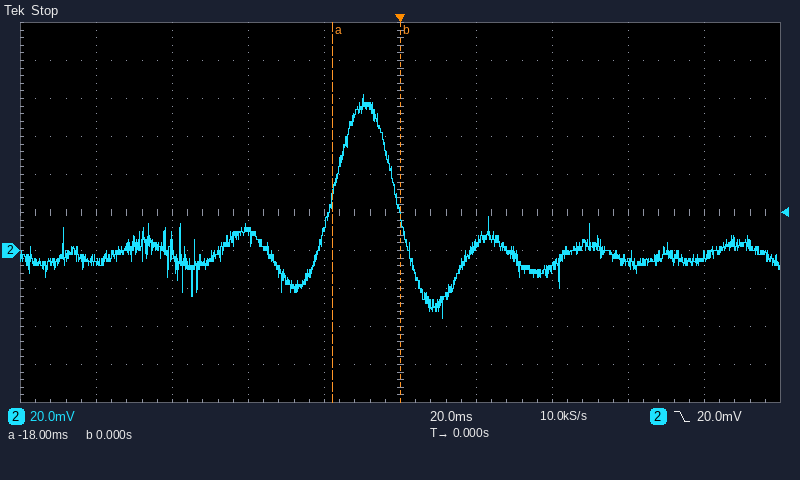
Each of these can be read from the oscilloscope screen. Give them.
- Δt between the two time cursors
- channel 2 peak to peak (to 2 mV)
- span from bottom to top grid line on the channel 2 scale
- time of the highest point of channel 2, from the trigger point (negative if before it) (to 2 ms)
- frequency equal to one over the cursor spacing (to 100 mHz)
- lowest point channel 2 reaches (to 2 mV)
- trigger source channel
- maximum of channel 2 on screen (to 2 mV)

18 ms
118 mV
200 mV
-10 ms
55.6 Hz
-36 mV
channel 2
82 mV
